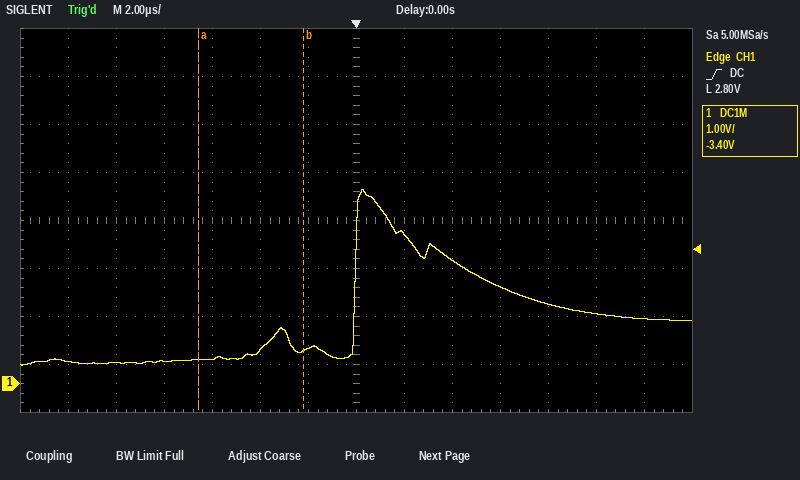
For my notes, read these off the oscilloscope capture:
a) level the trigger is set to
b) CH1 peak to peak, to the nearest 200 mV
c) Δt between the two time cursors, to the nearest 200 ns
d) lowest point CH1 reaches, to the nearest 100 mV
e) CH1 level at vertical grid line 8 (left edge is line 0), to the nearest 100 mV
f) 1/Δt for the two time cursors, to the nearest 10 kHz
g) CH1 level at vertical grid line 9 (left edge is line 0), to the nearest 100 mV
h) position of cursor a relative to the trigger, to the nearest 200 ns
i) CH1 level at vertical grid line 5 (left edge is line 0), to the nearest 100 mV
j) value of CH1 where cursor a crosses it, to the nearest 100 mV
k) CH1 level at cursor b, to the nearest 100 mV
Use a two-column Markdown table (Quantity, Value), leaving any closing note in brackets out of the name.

| Quantity | Value |
|---|---|
| level the trigger is set to | 2.80 V |
| CH1 peak to peak, to the nearest 200 mV | 3.6 V |
| Δt between the two time cursors, to the nearest 200 ns | 4.4 µs |
| lowest point CH1 reaches, to the nearest 100 mV | 400 mV |
| CH1 level at vertical grid line 8 (left edge is line 0), to the nearest 100 mV | 3.1 V |
| 1/Δt for the two time cursors, to the nearest 10 kHz | 230 kHz |
| CH1 level at vertical grid line 9 (left edge is line 0), to the nearest 100 mV | 2.6 V |
| position of cursor a relative to the trigger, to the nearest 200 ns | -6.6 µs |
| CH1 level at vertical grid line 5 (left edge is line 0), to the nearest 100 mV | 700 mV |
| value of CH1 where cursor a crosses it, to the nearest 100 mV | 500 mV |
| CH1 level at cursor b, to the nearest 100 mV | 700 mV |
